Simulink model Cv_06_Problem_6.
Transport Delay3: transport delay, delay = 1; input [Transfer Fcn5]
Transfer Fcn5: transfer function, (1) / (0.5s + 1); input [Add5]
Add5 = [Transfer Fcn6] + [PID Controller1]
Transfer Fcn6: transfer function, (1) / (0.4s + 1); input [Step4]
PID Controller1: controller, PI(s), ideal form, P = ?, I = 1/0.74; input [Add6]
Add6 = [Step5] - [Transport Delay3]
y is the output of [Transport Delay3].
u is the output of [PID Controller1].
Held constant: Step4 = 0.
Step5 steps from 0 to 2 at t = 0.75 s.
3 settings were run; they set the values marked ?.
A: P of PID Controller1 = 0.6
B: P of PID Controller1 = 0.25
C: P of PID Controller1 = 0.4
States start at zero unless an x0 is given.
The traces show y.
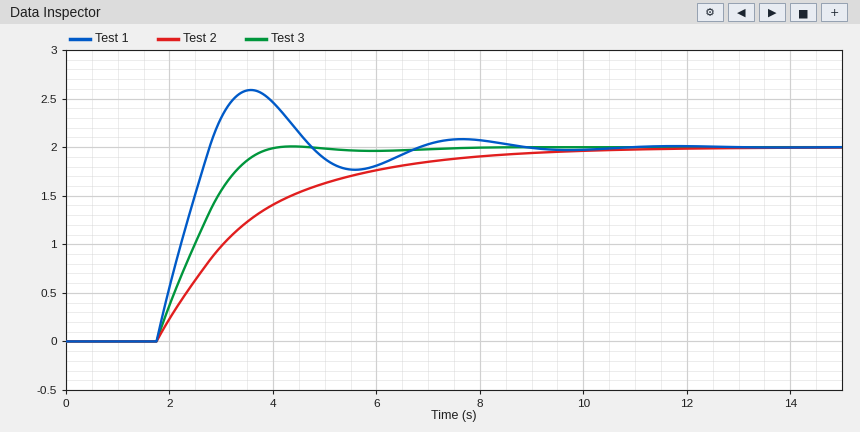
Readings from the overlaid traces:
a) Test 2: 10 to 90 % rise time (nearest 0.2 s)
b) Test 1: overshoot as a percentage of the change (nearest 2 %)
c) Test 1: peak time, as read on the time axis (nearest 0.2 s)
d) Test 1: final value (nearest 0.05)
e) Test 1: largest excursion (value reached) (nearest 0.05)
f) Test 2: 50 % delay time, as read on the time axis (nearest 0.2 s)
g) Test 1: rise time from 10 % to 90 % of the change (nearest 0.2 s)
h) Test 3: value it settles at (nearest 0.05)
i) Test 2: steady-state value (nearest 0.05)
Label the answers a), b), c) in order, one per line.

a) 4.4 s
b) 30 %
c) 3.6 s
d) 2.00
e) 2.60
f) 3.0 s
g) 0.8 s
h) 2.00
i) 2.00
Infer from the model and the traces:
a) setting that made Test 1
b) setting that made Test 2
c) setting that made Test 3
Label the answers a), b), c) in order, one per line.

a) A
b) B
c) C
